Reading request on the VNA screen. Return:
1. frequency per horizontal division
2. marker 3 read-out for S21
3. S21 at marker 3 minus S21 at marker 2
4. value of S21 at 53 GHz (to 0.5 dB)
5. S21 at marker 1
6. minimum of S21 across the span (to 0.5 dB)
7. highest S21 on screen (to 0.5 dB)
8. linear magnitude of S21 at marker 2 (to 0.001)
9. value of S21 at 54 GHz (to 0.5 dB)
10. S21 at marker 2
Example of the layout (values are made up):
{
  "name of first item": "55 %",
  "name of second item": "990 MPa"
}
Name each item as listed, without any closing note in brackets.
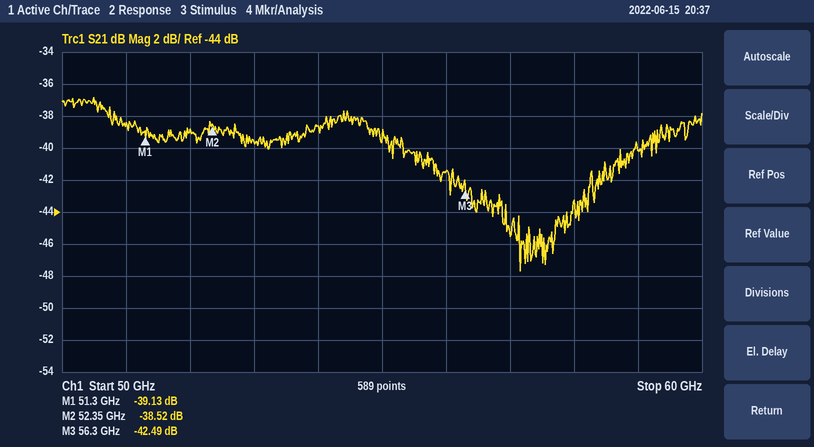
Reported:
{
  "frequency per horizontal division": "1 GHz",
  "marker 3 read-out for S21": "-42.49 dB",
  "S21 at marker 3 minus S21 at marker 2": "-3.97 dB",
  "value of S21 at 53 GHz": "-39.5 dB",
  "S21 at marker 1": "-39.13 dB",
  "minimum of S21 across the span": "-47.5 dB",
  "highest S21 on screen": "-37.0 dB",
  "linear magnitude of S21 at marker 2": "0.012",
  "value of S21 at 54 GHz": "-38.5 dB",
  "S21 at marker 2": "-38.52 dB"
}
